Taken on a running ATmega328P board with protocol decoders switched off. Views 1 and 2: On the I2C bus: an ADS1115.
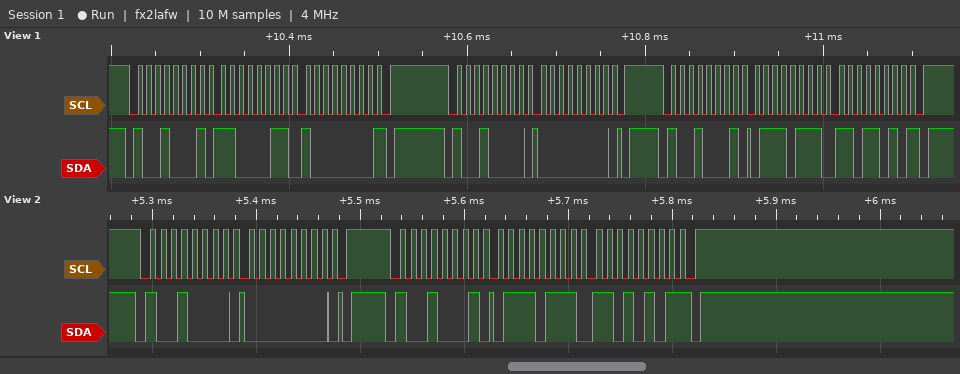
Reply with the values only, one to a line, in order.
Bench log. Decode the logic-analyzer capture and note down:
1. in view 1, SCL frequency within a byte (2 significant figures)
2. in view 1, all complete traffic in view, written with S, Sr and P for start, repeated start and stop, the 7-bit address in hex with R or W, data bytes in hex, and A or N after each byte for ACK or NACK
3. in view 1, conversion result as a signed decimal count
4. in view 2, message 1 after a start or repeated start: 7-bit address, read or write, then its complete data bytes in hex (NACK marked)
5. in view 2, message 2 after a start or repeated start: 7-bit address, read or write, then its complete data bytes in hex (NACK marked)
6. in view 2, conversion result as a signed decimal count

100 kHz
S 48R A C3 A 80 N P S 48W A 00 A P S 48R A 77 A DA N P
30682
0x48 write: 00
0x48 read: 77 D5 NACK
30677
